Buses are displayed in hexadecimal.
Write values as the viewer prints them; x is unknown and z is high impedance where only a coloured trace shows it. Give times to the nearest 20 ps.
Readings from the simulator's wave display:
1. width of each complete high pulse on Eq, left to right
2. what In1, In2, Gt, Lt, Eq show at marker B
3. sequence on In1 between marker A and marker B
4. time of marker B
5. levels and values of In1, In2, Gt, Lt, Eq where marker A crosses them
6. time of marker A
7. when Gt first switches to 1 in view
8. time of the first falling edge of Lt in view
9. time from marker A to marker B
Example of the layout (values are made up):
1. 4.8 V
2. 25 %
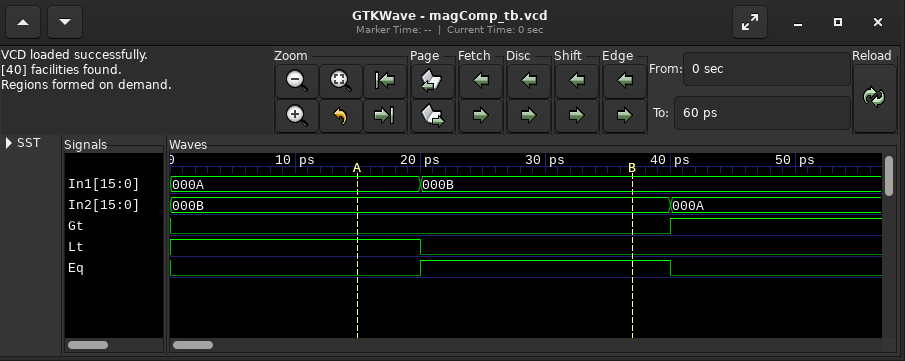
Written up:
1. 20 ps
2. In1=000B, In2=000B, Gt=0, Lt=0, Eq=1
3. 000A, 000B
4. 40 ps
5. In1=000A, In2=000B, Gt=0, Lt=1, Eq=0
6. 20 ps
7. 40 ps
8. 20 ps
9. 20 ps
